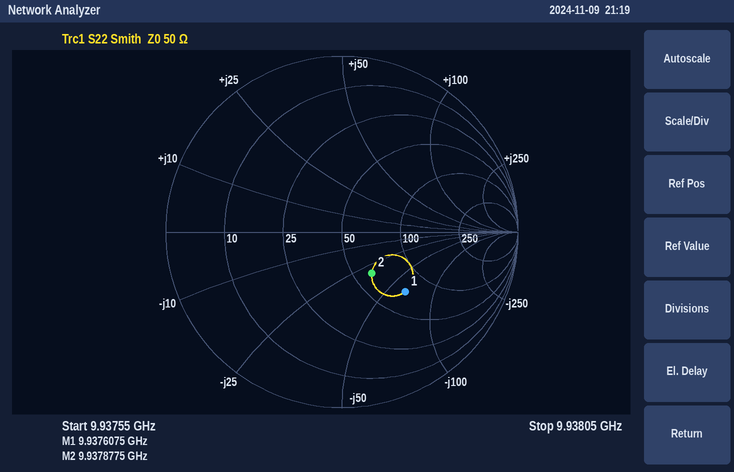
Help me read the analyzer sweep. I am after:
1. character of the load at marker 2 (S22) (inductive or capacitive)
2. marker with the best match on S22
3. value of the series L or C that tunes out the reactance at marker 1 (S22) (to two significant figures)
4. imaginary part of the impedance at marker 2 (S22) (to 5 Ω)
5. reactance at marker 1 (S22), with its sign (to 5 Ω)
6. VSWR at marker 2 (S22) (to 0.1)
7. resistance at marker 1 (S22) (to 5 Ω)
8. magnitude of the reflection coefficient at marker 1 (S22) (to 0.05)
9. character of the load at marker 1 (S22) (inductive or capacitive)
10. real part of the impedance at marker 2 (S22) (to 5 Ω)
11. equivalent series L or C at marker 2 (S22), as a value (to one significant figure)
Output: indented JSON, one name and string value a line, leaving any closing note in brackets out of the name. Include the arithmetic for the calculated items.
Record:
{
  "character of the load at marker 2 (S22)": "capacitive",
  "marker with the best match on S22": "marker 2",
  "value of the series L or C that tunes out the reactance at marker 1 (S22)": "L = 65 Ω/(2π × 9.9376075 GHz) ≈ 1.0 nH",
  "imaginary part of the impedance at marker 2 (S22)": "-30 Ω",
  "reactance at marker 1 (S22), with its sign": "-65 Ω",
  "VSWR at marker 2 (S22)": "1.8",
  "resistance at marker 1 (S22)": "70 Ω",
  "magnitude of the reflection coefficient at marker 1 (S22)": "0.50",
  "character of the load at marker 1 (S22)": "capacitive",
  "real part of the impedance at marker 2 (S22)": "60 Ω",
  "equivalent series L or C at marker 2 (S22), as a value": "C = 1/(2π × 9.9378775 GHz × 30 Ω) ≈ 534 fF, so 500 fF to one significant figure"
}
